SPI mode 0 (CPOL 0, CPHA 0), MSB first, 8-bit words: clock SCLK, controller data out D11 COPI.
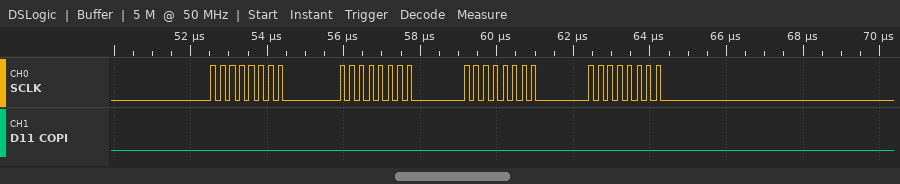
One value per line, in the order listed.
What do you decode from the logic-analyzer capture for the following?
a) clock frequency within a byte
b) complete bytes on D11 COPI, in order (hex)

4 MHz
00 00 00 00
